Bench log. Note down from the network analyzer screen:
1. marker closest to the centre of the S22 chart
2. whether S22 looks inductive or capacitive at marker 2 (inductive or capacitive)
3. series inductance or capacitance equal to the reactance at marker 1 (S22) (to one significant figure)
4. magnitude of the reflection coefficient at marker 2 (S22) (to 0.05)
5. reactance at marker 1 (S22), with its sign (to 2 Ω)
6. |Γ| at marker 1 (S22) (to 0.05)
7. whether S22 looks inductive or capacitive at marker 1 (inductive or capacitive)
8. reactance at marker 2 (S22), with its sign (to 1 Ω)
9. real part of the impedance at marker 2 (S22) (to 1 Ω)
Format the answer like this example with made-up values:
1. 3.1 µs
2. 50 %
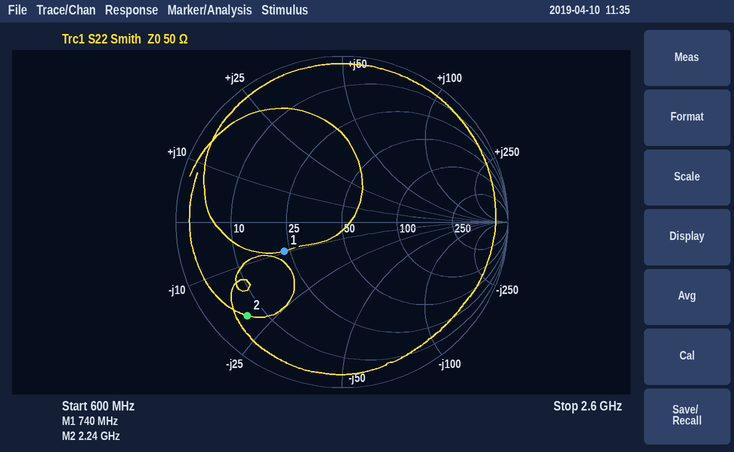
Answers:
1. marker 1
2. capacitive
3. 20 pF
4. 0.80
5. -10 Ω
6. 0.40
7. capacitive
8. -20 Ω
9. 6 Ω
